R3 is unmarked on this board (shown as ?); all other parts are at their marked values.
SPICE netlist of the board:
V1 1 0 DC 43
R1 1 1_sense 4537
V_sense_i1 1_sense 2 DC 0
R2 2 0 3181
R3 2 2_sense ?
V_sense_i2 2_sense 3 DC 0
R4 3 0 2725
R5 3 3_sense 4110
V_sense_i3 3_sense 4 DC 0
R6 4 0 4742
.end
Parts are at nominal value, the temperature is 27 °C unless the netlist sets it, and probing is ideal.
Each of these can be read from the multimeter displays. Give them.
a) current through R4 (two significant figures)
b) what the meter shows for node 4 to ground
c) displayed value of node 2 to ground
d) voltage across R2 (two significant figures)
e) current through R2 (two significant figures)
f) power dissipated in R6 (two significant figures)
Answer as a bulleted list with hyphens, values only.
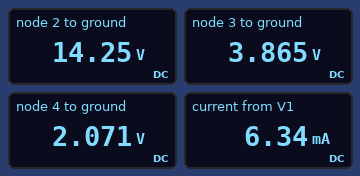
- 1.4 mA
- 2.071 V
- 14.25 V
- 14 V
- 4.5 mA
- 900 µW
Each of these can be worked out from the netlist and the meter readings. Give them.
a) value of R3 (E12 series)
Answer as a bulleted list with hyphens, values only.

- 5.6 kΩ
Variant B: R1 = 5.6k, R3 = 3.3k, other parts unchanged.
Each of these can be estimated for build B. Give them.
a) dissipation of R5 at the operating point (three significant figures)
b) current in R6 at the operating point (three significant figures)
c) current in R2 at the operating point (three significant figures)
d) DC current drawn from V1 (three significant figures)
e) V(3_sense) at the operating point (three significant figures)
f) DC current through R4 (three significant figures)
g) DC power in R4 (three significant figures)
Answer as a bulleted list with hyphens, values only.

- 1.01 mW
- 495 µA
- 3.56 mA
- 5.66 mA
- 2.35 V
- 1.61 mA
- 7.04 mW
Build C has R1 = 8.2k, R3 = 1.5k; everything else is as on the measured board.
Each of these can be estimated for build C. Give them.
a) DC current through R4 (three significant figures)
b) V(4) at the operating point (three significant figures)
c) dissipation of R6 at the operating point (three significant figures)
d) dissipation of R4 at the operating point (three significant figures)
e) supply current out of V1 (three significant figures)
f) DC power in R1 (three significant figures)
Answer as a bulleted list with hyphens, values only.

- 1.56 mA
- 2.28 V
- 1.10 mW
- 6.67 mW
- 4.35 mA
- 155 mW
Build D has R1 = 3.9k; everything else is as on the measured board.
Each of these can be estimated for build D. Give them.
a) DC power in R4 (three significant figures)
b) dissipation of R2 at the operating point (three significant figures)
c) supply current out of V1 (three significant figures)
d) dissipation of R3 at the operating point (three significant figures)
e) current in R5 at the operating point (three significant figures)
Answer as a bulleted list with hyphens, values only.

- 6.68 mW
- 77.8 mW
- 6.99 mA
- 23.5 mW
- 482 µA
